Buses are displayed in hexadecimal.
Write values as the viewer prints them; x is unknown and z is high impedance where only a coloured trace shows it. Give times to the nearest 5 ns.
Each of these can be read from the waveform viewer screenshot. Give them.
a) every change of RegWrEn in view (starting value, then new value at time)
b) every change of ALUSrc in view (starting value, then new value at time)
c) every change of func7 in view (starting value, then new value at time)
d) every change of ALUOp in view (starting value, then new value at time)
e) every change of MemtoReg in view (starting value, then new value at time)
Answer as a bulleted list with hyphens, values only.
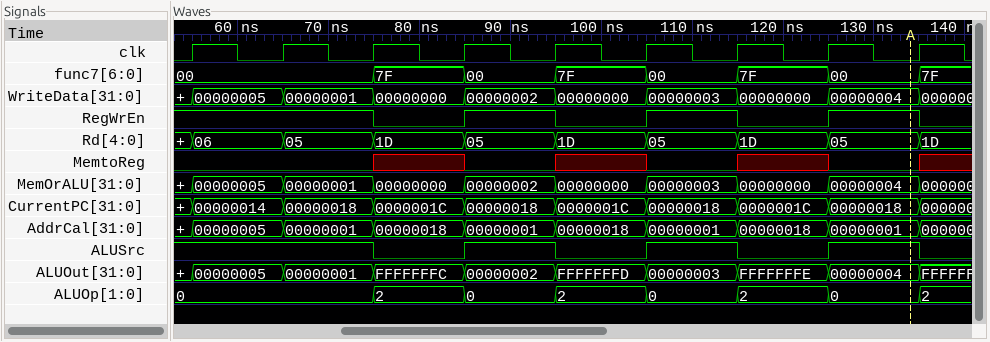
- 1, 0 at 75 ns, 1 at 85 ns, 0 at 95 ns, 1 at 105 ns, 0 at 115 ns, 1 at 125 ns, 0 at 135 ns
- 1, 0 at 75 ns, 1 at 85 ns, 0 at 95 ns, 1 at 105 ns, 0 at 115 ns, 1 at 125 ns, 0 at 135 ns
- 00, 7F at 75 ns, 00 at 85 ns, 7F at 95 ns, 00 at 105 ns, 7F at 115 ns, 00 at 125 ns, 7F at 135 ns
- 0, 2 at 75 ns, 0 at 85 ns, 2 at 95 ns, 0 at 105 ns, 2 at 115 ns, 0 at 125 ns, 2 at 135 ns
- 0, x at 75 ns, 0 at 85 ns, x at 95 ns, 0 at 105 ns, x at 115 ns, 0 at 125 ns, x at 135 ns
